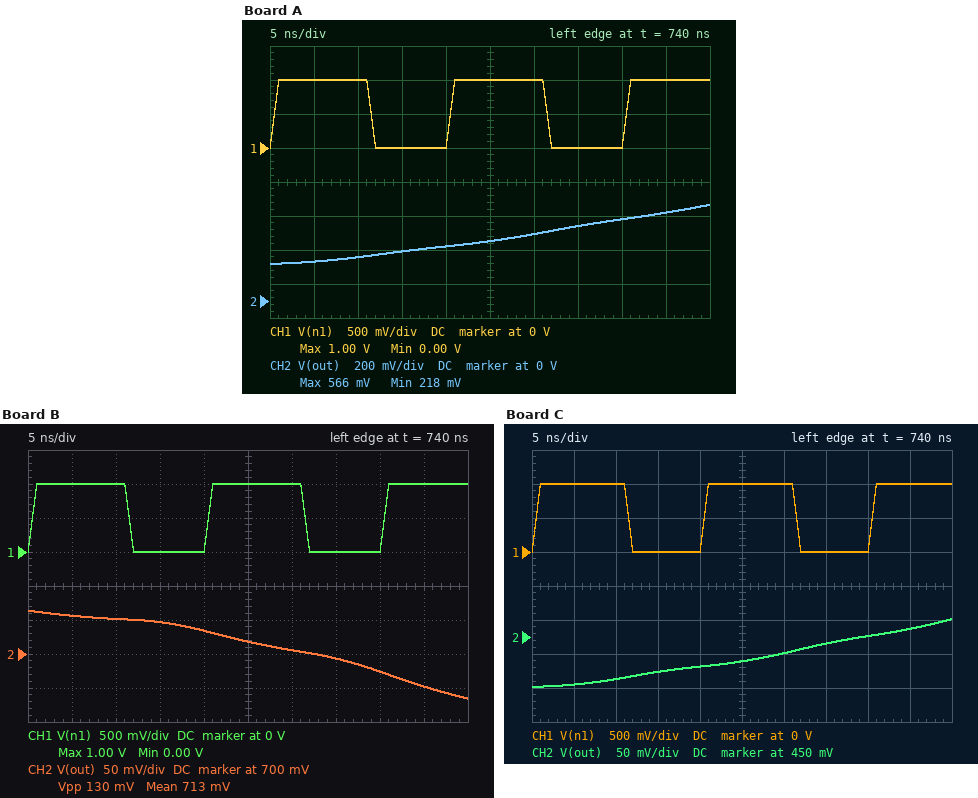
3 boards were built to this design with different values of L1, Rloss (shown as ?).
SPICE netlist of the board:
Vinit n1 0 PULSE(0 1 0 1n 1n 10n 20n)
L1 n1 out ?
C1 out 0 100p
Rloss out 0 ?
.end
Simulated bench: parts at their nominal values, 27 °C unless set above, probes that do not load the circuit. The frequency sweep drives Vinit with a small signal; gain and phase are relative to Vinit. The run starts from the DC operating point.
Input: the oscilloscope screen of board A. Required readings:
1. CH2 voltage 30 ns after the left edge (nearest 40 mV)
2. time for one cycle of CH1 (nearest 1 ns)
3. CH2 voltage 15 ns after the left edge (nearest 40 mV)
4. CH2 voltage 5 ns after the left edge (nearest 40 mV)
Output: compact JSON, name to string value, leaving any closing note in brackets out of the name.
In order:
{"CH2 voltage 30 ns after the left edge": "400 mV", "time for one cycle of CH1": "20 ns", "CH2 voltage 15 ns after the left edge": "280 mV", "CH2 voltage 5 ns after the left edge": "240 mV"}
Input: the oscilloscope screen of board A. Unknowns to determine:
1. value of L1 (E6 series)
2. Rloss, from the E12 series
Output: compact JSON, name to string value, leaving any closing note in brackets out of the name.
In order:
{"value of L1": "15 µH", "Rloss, from the E12 series": "8.2 kΩ"}
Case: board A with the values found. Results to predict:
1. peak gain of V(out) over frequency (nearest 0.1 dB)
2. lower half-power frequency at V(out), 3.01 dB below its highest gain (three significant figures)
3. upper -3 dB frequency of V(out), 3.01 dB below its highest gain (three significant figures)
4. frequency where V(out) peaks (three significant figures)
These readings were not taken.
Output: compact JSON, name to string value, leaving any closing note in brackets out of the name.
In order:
{"peak gain of V(out) over frequency": "26.5 dB", "lower half-power frequency at V(out), 3.01 dB below its highest gain": "4.01 MHz", "upper -3 dB frequency of V(out), 3.01 dB below its highest gain": "4.20 MHz", "frequency where V(out) peaks": "4.11 MHz"}
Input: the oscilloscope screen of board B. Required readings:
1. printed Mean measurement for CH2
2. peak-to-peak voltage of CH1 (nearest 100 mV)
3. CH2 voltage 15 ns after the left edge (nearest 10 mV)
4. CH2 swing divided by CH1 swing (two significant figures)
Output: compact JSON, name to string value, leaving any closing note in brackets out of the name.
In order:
{"printed Mean measurement for CH2": "713 mV", "peak-to-peak voltage of CH1": "1.0 V", "CH2 voltage 15 ns after the left edge": "750 mV", "CH2 swing divided by CH1 swing": "0.13"}
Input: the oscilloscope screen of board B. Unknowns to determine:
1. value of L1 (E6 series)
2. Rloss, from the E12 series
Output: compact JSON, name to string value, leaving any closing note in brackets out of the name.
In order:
{"value of L1": "22 µH", "Rloss, from the E12 series": "3.9 kΩ"}
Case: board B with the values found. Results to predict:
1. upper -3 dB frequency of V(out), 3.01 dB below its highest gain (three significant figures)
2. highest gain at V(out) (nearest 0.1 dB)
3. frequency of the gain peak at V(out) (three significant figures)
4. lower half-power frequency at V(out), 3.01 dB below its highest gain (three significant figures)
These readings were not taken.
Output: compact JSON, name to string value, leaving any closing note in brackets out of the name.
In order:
{"upper -3 dB frequency of V(out), 3.01 dB below its highest gain": "3.58 MHz", "highest gain at V(out)": "18.4 dB", "frequency of the gain peak at V(out)": "3.38 MHz", "lower half-power frequency at V(out), 3.01 dB below its highest gain": "3.17 MHz"}
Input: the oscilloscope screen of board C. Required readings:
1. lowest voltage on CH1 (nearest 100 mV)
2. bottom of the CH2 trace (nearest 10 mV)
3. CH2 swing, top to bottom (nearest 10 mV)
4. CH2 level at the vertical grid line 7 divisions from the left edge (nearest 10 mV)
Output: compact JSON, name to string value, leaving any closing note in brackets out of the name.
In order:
{"lowest voltage on CH1": "0 V", "bottom of the CH2 trace": "380 mV", "CH2 swing, top to bottom": "100 mV", "CH2 level at the vertical grid line 7 divisions from the left edge": "440 mV"}
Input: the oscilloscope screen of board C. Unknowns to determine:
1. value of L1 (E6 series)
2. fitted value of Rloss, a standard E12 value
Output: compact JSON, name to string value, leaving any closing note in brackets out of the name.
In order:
{"value of L1": "33 µH", "fitted value of Rloss, a standard E12 value": "3.3 kΩ"}
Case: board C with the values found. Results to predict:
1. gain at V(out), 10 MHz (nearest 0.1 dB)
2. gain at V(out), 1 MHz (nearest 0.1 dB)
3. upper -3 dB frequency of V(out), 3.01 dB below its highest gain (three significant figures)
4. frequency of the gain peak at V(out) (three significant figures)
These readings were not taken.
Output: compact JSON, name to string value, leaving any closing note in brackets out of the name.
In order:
{"gain at V(out), 10 MHz": "-21.6 dB", "gain at V(out), 1 MHz": "1.2 dB", "upper -3 dB frequency of V(out), 3.01 dB below its highest gain": "2.98 MHz", "frequency of the gain peak at V(out)": "2.75 MHz"}
